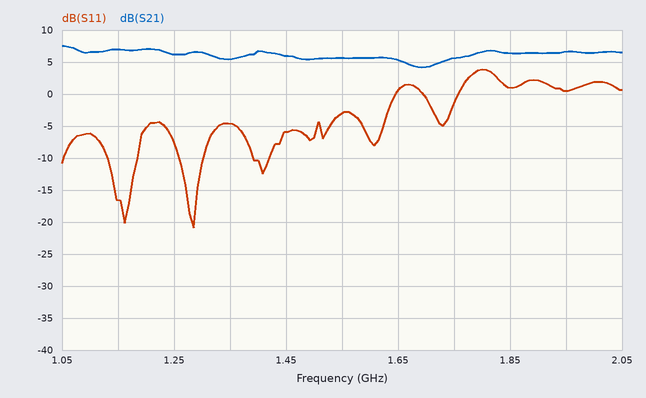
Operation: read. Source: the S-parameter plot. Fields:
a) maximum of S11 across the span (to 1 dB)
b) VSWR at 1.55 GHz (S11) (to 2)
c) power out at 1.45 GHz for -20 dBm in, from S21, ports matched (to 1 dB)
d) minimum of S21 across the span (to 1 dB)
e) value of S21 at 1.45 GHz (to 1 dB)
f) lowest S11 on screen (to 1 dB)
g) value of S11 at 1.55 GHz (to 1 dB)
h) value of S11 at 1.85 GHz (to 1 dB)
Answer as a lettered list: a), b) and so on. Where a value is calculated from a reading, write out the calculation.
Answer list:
a) 4 dB
b) |Γ| = 10^(-3/20) = 0.7079; VSWR = (1 + 0.7079)/(1 − 0.7079) ≈ 6
c) -20 dBm + (6 dB) = -14 dBm
d) 4 dB
e) 6 dB
f) -21 dB
g) -3 dB
h) 1 dB
